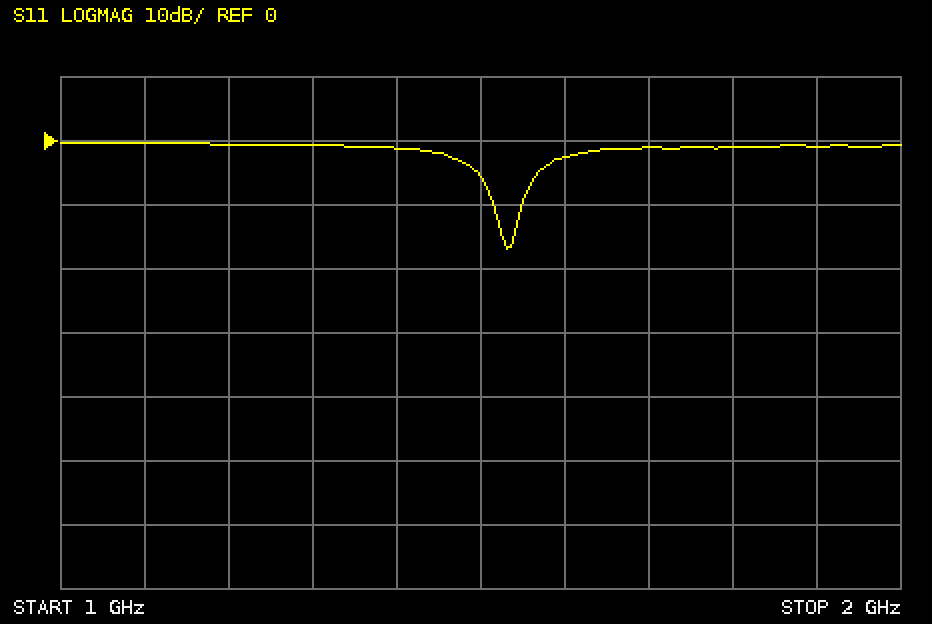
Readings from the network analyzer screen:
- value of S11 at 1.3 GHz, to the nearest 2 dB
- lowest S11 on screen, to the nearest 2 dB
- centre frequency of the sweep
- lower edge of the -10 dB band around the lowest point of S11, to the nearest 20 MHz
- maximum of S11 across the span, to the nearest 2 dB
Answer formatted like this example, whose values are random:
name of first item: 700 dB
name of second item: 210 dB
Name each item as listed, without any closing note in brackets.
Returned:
value of S11 at 1.3 GHz, to the nearest 2 dB: 0 dB
lowest S11 on screen, to the nearest 2 dB: -16 dB
centre frequency of the sweep: 1.5 GHz
lower edge of the -10 dB band around the lowest point of S11, to the nearest 20 MHz: 1.52 GHz
maximum of S11 across the span, to the nearest 2 dB: 0 dB
